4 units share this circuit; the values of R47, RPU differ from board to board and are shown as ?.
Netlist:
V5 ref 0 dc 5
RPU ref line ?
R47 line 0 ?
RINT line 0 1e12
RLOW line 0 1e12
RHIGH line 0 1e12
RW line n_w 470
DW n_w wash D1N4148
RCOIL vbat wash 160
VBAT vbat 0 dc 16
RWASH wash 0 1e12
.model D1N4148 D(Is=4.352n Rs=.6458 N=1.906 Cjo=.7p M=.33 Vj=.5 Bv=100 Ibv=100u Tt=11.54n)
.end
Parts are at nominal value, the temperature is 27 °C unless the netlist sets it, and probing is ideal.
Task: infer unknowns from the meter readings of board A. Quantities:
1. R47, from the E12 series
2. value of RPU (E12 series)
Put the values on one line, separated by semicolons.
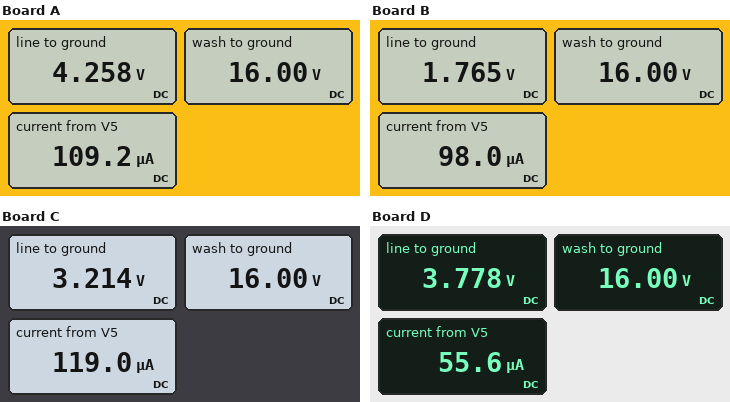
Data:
39 kΩ; 6.8 kΩ
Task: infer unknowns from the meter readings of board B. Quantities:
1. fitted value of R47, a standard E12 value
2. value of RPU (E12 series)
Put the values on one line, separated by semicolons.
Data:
18 kΩ; 33 kΩ
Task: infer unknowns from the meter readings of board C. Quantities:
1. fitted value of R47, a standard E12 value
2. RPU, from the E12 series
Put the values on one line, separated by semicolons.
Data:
27 kΩ; 15 kΩ
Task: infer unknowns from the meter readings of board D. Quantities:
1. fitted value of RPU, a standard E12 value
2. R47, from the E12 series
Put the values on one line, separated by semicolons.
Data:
22 kΩ; 68 kΩ
